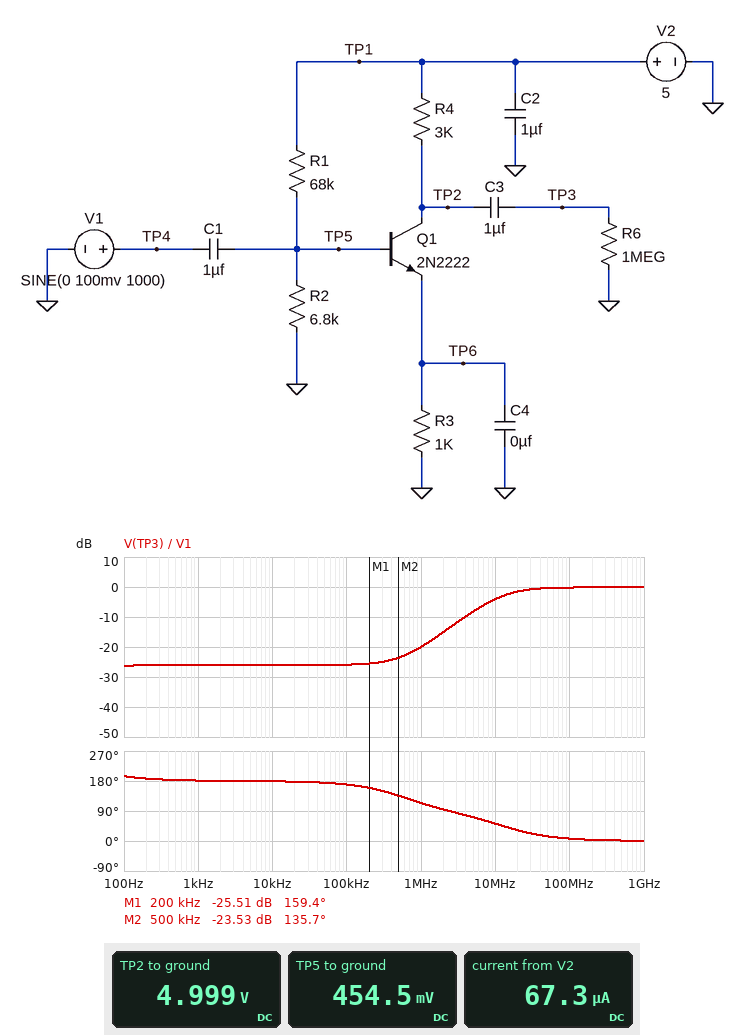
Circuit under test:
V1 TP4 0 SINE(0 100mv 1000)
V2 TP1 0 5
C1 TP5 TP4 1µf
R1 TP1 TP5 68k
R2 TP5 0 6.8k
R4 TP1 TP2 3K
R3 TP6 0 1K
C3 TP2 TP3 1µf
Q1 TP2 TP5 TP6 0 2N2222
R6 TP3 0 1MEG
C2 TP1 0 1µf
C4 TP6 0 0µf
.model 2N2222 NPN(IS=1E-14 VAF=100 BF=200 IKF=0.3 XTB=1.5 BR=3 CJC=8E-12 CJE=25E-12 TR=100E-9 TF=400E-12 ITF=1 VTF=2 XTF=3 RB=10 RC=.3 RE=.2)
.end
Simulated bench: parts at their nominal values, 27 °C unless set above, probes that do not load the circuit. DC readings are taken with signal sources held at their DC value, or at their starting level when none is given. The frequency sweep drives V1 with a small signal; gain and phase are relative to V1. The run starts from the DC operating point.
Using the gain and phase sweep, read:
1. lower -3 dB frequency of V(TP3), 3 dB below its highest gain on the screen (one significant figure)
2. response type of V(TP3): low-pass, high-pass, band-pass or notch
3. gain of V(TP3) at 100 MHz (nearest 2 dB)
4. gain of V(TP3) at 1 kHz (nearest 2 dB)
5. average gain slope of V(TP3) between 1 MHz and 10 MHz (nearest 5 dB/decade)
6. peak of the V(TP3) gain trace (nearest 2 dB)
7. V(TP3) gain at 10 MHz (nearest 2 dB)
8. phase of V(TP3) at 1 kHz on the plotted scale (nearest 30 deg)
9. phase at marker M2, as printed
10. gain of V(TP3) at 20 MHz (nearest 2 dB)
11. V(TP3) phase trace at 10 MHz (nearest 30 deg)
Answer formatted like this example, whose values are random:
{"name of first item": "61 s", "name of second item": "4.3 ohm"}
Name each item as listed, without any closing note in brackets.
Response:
{"lower -3 dB frequency of V(TP3), 3 dB below its highest gain on the screen": "10 MHz", "response type of V(TP3): low-pass, high-pass, band-pass or notch": "high-pass", "gain of V(TP3) at 100 MHz": "0 dB", "gain of V(TP3) at 1 kHz": "-26 dB", "average gain slope of V(TP3) between 1 MHz and 10 MHz": "15 dB/decade", "peak of the V(TP3) gain trace": "0 dB", "V(TP3) gain at 10 MHz": "-4 dB", "phase of V(TP3) at 1 kHz on the plotted scale": "180 deg", "phase at marker M2, as printed": "135.7 deg", "gain of V(TP3) at 20 MHz": "-2 dB", "V(TP3) phase trace at 10 MHz": "60 deg"}
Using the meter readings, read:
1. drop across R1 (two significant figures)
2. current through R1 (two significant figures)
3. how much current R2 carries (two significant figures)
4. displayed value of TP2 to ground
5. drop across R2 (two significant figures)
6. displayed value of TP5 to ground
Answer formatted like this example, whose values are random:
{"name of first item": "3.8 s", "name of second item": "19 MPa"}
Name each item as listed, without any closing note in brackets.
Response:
{"drop across R1": "4.5 V", "current through R1": "67 µA", "how much current R2 carries": "67 µA", "displayed value of TP2 to ground": "4.999 V", "drop across R2": "450 mV", "displayed value of TP5 to ground": "454.5 mV"}
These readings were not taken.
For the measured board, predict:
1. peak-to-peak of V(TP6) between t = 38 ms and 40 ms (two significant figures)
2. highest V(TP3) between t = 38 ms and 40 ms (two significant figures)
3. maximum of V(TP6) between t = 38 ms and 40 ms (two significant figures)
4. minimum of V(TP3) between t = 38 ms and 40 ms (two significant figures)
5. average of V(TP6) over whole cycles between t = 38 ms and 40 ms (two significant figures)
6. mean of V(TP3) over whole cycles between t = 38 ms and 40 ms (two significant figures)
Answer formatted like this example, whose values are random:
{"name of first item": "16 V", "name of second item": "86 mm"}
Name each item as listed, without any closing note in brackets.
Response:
{"peak-to-peak of V(TP6) between t = 38 ms and 40 ms": "13 mV", "highest V(TP3) between t = 38 ms and 40 ms": "1.6 mV", "maximum of V(TP6) between t = 38 ms and 40 ms": "13 mV", "minimum of V(TP3) between t = 38 ms and 40 ms": "-37 mV", "average of V(TP6) over whole cycles between t = 38 ms and 40 ms": "3.1 mV", "mean of V(TP3) over whole cycles between t = 38 ms and 40 ms": "-7.7 mV"}
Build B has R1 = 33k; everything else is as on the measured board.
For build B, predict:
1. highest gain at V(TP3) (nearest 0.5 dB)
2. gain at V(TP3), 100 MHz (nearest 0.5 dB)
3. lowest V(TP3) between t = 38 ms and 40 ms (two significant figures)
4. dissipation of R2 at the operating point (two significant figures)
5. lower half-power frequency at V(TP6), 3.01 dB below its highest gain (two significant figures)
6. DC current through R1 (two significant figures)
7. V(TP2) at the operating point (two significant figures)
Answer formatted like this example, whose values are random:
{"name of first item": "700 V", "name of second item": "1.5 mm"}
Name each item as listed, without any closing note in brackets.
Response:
{"highest gain at V(TP3)": "8.5 dB", "gain at V(TP3), 100 MHz": "0.5 dB", "lowest V(TP3) between t = 38 ms and 40 ms": "-270 mV", "dissipation of R2 at the operating point": "110 µW", "lower half-power frequency at V(TP6), 3.01 dB below its highest gain": "36 Hz", "DC current through R1": "130 µA", "V(TP2) at the operating point": "4.3 V"}
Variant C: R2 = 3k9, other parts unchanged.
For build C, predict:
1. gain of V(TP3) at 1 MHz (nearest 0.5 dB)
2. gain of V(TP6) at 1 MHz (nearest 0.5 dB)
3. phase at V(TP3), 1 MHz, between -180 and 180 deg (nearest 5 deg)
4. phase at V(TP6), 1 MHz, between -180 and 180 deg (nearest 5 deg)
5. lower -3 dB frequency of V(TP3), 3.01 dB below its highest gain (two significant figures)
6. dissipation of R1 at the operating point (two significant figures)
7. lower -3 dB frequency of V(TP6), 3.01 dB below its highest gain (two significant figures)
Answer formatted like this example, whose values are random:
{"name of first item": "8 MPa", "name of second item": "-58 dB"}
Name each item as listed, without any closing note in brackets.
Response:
{"gain of V(TP3) at 1 MHz": "-22.0 dB", "gain of V(TP6) at 1 MHz": "-15.0 dB", "phase at V(TP3), 1 MHz, between -180 and 180 deg": "85 deg", "phase at V(TP6), 1 MHz, between -180 and 180 deg": "80 deg", "lower -3 dB frequency of V(TP3), 3.01 dB below its highest gain": "13 MHz", "dissipation of R1 at the operating point": "330 µW", "lower -3 dB frequency of V(TP6), 3.01 dB below its highest gain": "5.4 MHz"}
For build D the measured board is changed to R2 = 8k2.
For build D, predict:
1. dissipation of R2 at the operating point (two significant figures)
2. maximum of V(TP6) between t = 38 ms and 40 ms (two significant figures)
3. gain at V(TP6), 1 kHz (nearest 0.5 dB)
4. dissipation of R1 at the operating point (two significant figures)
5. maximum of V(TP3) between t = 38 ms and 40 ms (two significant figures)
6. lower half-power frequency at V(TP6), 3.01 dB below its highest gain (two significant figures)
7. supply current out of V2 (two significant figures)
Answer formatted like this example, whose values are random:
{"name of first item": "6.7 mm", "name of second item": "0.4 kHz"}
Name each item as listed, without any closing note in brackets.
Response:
{"dissipation of R2 at the operating point": "35 µW", "maximum of V(TP6) between t = 38 ms and 40 ms": "57 mV", "gain at V(TP6), 1 kHz": "-12.5 dB", "dissipation of R1 at the operating point": "290 µW", "maximum of V(TP3) between t = 38 ms and 40 ms": "25 mV", "lower half-power frequency at V(TP6), 3.01 dB below its highest gain": "5.4 MHz", "supply current out of V2": "74 µA"}
